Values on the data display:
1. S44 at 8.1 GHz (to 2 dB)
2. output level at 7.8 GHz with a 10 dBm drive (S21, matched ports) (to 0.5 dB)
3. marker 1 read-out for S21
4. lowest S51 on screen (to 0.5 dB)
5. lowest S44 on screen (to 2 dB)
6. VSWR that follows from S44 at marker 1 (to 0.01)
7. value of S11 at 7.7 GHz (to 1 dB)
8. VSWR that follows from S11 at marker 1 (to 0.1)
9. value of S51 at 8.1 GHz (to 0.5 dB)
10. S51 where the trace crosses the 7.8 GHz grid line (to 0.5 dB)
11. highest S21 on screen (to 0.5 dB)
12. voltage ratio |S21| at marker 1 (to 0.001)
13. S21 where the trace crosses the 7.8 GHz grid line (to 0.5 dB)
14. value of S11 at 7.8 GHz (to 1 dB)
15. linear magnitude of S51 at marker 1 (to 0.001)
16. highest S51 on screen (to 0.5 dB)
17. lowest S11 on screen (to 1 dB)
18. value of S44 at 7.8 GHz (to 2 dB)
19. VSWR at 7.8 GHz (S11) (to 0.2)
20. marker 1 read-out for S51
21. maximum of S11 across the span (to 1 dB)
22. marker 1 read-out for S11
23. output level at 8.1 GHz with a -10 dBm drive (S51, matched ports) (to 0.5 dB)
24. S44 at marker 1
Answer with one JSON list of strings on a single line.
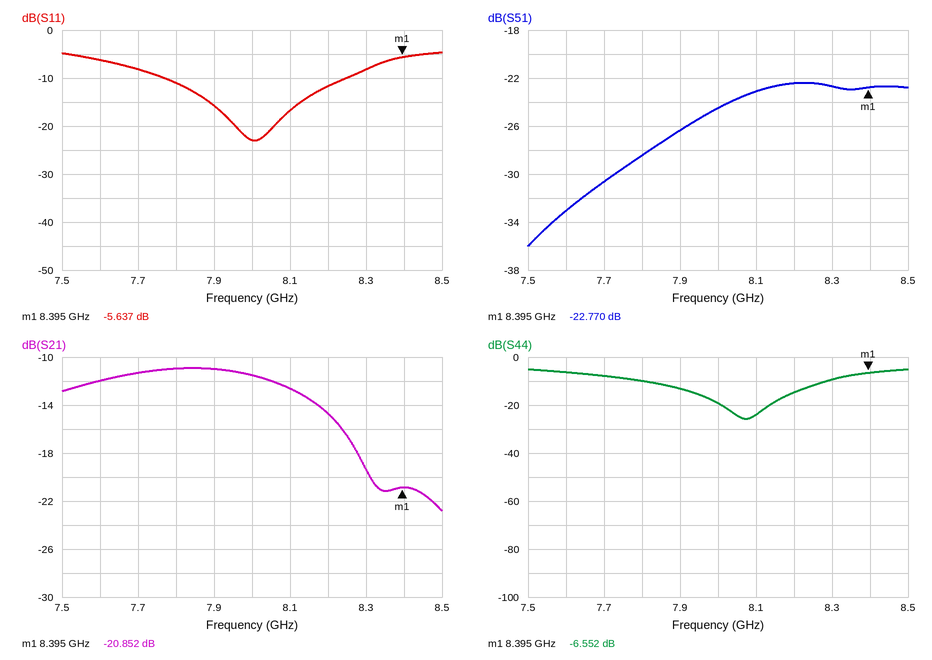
["-24 dB", "-1.0 dBm", "-20.852 dB", "-36.0 dB", "-26 dB", "2.78", "-8 dB", "3.2", "-23.0 dB", "-28.5 dB", "-11.0 dB", "0.091", "-11.0 dB", "-11 dB", "0.073", "-22.5 dB", "-23 dB", "-10 dB", "1.8", "-22.770 dB", "-5 dB", "-5.637 dB", "-33.0 dBm", "-6.552 dB"]
